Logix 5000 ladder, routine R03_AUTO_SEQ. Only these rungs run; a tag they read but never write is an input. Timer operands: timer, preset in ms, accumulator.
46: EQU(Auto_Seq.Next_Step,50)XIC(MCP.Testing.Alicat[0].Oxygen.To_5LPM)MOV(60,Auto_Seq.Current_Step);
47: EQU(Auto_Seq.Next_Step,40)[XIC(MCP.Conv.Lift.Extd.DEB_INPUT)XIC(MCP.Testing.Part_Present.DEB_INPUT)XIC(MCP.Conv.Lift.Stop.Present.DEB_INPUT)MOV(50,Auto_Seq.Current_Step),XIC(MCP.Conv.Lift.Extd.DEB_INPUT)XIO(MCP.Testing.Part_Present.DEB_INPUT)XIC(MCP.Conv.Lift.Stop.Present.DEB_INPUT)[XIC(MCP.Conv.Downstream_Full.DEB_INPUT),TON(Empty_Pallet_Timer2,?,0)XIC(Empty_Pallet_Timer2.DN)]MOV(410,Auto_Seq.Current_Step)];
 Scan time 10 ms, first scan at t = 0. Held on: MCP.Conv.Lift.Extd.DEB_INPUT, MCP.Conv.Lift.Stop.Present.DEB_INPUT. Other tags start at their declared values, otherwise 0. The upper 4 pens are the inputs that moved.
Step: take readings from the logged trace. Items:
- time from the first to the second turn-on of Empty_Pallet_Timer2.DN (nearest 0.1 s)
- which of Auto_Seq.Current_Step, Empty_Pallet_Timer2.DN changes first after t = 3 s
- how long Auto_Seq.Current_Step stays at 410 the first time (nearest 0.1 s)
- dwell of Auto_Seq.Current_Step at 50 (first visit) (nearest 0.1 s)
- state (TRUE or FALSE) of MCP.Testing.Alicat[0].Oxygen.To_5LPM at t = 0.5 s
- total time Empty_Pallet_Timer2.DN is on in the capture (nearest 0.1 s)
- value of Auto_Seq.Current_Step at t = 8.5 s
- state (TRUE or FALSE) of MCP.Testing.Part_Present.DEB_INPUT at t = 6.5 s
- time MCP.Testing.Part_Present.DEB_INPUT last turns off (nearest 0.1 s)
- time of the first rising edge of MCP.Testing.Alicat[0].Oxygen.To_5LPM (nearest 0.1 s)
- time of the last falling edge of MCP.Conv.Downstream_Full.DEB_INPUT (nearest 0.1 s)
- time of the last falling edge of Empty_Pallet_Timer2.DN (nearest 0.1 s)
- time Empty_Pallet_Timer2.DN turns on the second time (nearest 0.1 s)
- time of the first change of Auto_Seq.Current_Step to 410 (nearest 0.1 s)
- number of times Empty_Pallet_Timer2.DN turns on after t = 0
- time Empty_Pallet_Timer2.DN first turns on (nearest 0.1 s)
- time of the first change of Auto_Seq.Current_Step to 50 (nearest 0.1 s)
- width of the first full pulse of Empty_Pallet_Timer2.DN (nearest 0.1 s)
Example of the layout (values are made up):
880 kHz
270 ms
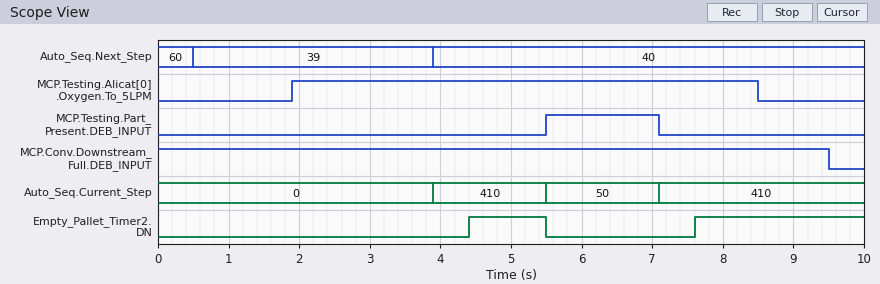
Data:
3.2 s
Auto_Seq.Current_Step
1.6 s
1.6 s
FALSE
3.5 s
410
TRUE
7.1 s
1.9 s
9.5 s
5.5 s
7.6 s
3.9 s
2
4.4 s
5.5 s
1.1 s
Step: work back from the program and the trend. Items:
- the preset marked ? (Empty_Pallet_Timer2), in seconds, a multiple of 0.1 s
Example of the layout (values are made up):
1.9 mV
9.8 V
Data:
0.5 s
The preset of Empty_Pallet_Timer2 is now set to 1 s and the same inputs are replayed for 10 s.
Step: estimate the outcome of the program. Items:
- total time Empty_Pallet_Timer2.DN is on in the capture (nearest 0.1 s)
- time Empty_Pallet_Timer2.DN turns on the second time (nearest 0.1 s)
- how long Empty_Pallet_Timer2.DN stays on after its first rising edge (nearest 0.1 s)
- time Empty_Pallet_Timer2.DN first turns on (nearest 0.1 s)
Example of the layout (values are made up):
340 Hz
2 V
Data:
2.5 s
8.1 s
0.6 s
4.9 s
